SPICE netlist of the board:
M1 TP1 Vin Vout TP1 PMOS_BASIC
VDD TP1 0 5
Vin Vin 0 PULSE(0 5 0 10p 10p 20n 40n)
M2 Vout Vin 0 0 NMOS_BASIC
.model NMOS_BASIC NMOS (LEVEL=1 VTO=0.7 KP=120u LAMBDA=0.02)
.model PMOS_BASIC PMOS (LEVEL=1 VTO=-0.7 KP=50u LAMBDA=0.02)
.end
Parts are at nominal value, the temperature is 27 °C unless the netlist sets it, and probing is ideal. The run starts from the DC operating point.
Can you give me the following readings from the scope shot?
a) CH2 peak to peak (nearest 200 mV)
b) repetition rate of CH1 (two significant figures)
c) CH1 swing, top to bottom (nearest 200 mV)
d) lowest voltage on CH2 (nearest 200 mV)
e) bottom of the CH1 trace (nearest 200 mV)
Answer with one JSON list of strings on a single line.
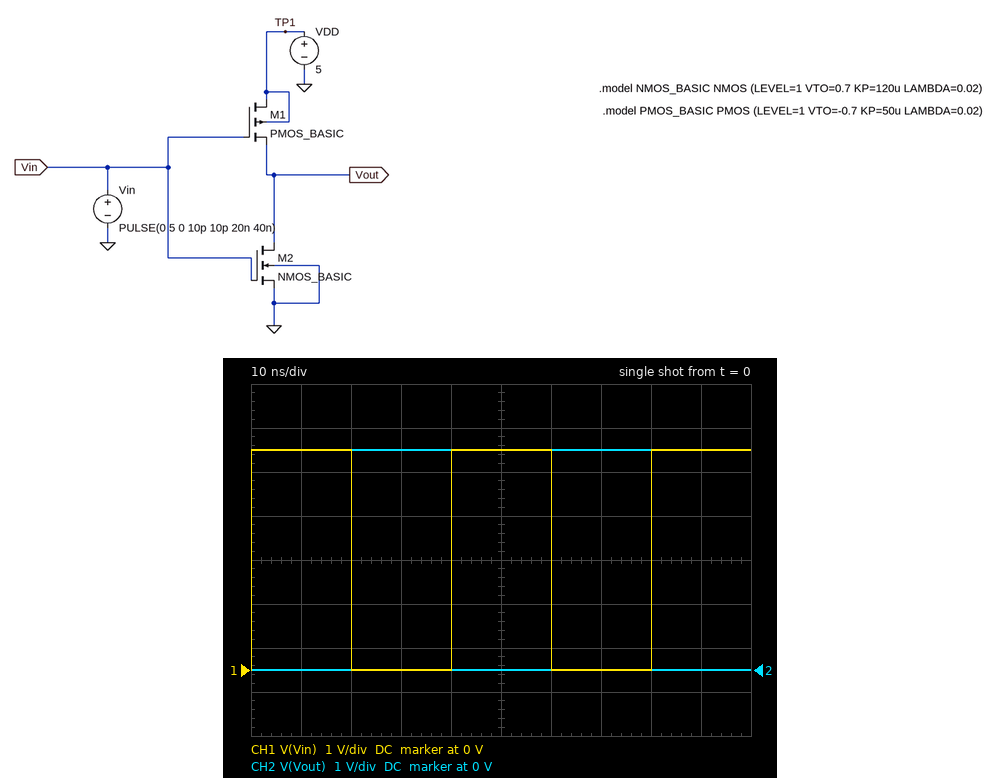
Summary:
["5.0 V", "25 MHz", "5.0 V", "0 V", "0 V"]
